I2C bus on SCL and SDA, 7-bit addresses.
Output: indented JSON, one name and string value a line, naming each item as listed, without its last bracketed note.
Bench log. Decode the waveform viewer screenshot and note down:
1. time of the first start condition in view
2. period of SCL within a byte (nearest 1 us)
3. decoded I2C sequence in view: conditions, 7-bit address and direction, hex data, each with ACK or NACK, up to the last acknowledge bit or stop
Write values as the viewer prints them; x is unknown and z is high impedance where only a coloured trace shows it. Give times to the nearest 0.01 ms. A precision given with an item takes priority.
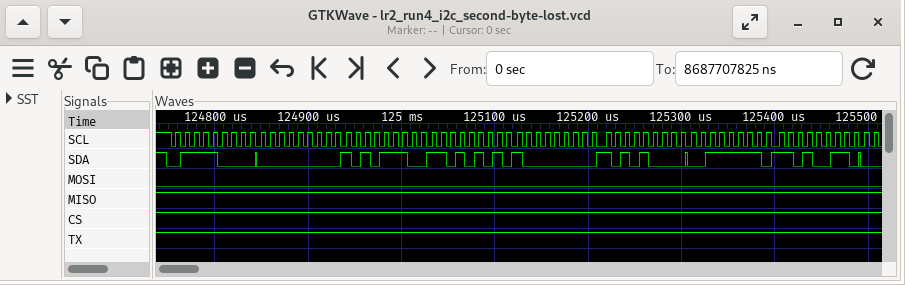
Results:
{
  "time of the first start condition in view": "124.75 ms",
  "period of SCL within a byte": "10 us",
  "decoded I2C sequence in view: conditions, 7-bit address and direction, hex data, each with ACK or NACK, up to the last acknowledge bit or stop": "start, address 3C write ACK, 00 ACK, AE ACK, D5 ACK, 80 ACK, A8 ACK, 3F ACK, D3 ACK"
}
